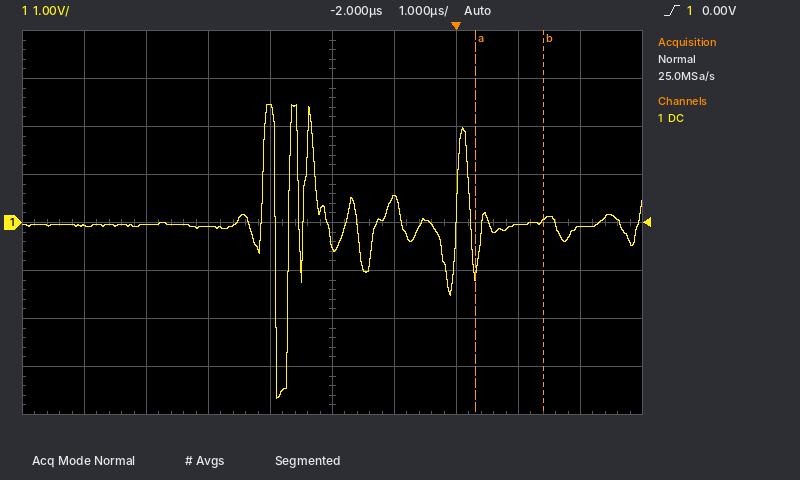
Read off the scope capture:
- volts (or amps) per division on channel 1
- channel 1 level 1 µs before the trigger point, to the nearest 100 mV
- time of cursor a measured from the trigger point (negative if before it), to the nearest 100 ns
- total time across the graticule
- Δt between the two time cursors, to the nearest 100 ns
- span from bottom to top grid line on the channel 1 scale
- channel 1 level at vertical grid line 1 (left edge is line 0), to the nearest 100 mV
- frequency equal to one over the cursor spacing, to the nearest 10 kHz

1 V
500 mV
+300 ns
10 µs
1.1 µs
8 V
-100 mV
910 kHz
